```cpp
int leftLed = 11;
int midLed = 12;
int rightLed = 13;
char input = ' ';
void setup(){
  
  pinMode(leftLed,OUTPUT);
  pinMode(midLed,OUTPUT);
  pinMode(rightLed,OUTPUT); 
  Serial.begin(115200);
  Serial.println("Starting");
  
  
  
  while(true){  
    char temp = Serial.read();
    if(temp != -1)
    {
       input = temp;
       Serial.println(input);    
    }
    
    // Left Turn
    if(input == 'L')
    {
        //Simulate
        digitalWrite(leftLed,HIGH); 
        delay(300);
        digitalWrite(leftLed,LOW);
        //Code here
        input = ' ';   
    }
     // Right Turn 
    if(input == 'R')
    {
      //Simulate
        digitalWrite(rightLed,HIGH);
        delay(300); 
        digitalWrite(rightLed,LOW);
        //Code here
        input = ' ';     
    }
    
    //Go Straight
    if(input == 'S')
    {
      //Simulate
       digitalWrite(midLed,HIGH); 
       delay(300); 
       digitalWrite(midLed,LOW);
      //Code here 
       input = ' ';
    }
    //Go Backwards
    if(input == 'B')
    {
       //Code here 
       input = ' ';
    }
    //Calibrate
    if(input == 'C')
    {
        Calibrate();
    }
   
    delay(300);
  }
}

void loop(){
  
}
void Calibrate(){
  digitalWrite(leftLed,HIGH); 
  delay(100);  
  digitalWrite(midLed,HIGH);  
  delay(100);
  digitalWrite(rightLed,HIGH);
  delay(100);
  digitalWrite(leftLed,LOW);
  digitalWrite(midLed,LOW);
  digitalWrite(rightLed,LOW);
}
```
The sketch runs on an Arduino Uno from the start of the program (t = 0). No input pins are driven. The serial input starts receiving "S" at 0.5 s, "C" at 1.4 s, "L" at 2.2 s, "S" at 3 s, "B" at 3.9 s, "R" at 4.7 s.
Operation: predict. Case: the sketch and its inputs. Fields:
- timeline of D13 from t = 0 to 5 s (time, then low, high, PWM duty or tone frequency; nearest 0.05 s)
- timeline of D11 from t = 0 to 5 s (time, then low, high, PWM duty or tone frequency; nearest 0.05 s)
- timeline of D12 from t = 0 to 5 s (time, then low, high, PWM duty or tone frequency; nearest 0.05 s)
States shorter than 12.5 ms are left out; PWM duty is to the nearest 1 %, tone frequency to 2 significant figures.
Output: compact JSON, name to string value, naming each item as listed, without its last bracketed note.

{"timeline of D13 from t = 0 to 5 s": "0 s low; 1.7 s high; 1.8 s low; 2.3 s high; 2.4 s low; 4.8 s high", "timeline of D11 from t = 0 to 5 s": "0 s low; 1.5 s high; 1.8 s low; 2.1 s high; 2.4 s low; 2.7 s high; 3 s low", "timeline of D12 from t = 0 to 5 s": "0 s low; 0.6 s high; 0.9 s low; 1.6 s high; 1.8 s low; 2.2 s high; 2.4 s low; 3.3 s high; 3.6 s low"}
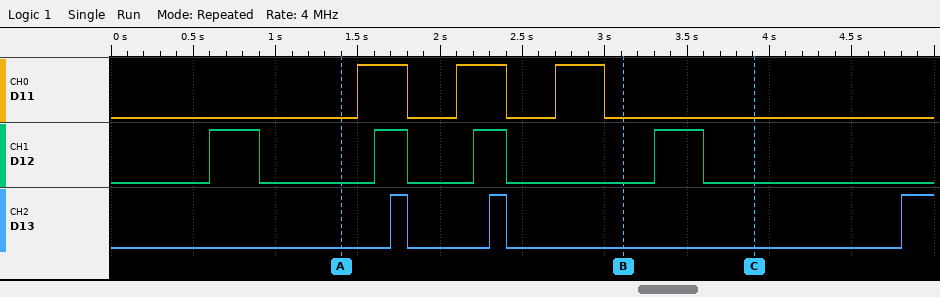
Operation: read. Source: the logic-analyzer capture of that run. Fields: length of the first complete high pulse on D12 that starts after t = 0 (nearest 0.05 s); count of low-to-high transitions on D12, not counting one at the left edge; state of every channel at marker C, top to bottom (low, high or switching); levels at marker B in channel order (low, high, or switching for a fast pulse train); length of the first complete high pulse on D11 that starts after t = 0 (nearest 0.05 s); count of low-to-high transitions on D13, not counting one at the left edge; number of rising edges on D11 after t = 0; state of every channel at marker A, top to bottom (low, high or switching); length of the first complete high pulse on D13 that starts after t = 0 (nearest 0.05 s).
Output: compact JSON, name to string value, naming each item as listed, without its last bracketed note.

{"length of the first complete high pulse on D12 that starts after t = 0": "0.30 s", "count of low-to-high transitions on D12, not counting one at the left edge": "4", "state of every channel at marker C, top to bottom": "D11 low, D12 low, D13 low", "levels at marker B in channel order": "D11 low, D12 low, D13 low", "length of the first complete high pulse on D11 that starts after t = 0": "0.30 s", "count of low-to-high transitions on D13, not counting one at the left edge": "3", "number of rising edges on D11 after t = 0": "3", "state of every channel at marker A, top to bottom": "D11 low, D12 low, D13 low", "length of the first complete high pulse on D13 that starts after t = 0": "0.10 s"}
